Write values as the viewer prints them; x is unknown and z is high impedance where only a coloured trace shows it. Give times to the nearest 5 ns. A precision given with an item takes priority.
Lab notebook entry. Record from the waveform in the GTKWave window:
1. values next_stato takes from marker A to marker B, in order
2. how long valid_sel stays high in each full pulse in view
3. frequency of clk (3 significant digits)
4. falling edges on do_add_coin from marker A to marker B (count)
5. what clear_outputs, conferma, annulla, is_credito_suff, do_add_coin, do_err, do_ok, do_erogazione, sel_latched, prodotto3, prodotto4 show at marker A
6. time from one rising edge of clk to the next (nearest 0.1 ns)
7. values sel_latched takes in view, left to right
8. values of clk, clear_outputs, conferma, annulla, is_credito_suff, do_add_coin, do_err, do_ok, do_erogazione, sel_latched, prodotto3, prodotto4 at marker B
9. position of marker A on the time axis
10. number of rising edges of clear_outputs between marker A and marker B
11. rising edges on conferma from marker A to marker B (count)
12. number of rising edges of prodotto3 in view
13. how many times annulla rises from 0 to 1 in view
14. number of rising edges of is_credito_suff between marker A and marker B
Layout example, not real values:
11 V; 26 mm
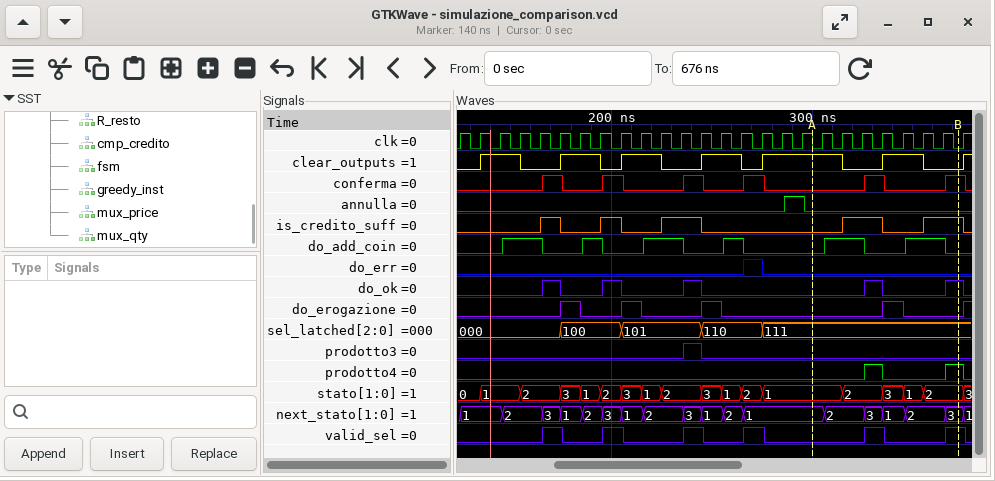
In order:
1, 2, 3, 1, 2, 3; 10 ns, 10 ns, 10 ns, 10 ns, 10 ns, 10 ns; 100 MHz; 2; clear_outputs=1, conferma=0, annulla=0, is_credito_suff=0, do_add_coin=0, do_err=0, do_ok=0, do_erogazione=0, sel_latched=111, prodotto3=0, prodotto4=0; 10 ns; 000, 100, 101, 110, 111; clk=0, clear_outputs=0, conferma=1, annulla=0, is_credito_suff=1, do_add_coin=0, do_err=0, do_ok=1, do_erogazione=0, sel_latched=111, prodotto3=0, prodotto4=1; 300 ns; 1; 2; 1; 1; 2
